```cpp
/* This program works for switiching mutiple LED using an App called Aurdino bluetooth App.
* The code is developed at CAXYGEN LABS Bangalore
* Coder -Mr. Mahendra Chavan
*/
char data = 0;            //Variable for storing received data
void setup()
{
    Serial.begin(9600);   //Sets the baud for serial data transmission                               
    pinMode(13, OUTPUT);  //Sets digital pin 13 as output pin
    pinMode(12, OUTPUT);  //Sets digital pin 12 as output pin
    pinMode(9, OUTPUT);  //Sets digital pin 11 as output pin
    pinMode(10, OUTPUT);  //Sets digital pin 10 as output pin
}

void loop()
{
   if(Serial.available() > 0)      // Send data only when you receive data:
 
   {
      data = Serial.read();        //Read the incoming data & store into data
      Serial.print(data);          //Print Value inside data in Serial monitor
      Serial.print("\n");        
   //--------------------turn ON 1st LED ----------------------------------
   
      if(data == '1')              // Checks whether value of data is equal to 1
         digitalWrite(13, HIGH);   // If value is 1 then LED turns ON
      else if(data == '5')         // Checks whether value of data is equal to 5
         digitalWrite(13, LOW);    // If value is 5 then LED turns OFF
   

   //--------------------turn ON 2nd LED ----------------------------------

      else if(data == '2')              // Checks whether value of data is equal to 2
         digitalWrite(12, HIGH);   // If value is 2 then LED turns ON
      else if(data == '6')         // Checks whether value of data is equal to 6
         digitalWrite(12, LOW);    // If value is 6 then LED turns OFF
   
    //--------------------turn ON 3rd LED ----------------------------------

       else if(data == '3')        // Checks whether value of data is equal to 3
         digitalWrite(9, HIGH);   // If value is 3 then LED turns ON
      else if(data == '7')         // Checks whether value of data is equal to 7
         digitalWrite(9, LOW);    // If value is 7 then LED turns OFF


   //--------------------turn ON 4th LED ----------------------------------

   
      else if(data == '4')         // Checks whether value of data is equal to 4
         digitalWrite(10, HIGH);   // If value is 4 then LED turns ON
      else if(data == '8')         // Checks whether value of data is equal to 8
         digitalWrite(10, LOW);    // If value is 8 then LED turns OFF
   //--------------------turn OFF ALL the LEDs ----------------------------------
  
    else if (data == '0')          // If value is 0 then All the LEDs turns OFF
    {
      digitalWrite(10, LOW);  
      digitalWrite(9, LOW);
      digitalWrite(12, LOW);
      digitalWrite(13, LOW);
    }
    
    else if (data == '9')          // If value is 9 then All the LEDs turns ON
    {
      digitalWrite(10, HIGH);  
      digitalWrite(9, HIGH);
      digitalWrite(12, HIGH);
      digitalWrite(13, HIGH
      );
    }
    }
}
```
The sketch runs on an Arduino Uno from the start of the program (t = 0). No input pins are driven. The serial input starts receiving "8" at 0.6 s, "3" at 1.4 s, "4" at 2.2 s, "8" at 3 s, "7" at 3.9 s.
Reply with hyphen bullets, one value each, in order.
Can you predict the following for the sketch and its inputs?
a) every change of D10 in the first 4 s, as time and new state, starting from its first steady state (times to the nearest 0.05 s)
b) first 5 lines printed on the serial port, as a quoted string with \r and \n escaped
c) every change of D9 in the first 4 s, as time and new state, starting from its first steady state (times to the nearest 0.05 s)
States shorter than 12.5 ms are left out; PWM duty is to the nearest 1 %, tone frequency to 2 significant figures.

- 0 s low; 2.2 s high; 3 s low
- "8\n3\n4\n8\n7\n"
- 0 s low; 1.4 s high; 3.9 s low
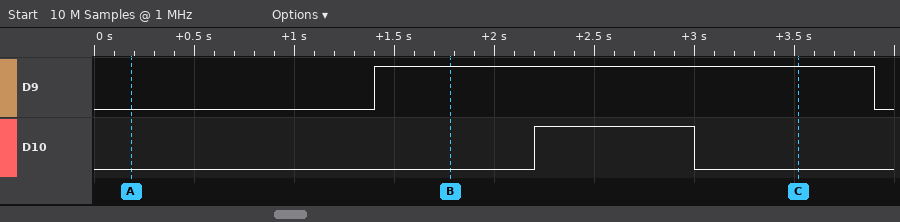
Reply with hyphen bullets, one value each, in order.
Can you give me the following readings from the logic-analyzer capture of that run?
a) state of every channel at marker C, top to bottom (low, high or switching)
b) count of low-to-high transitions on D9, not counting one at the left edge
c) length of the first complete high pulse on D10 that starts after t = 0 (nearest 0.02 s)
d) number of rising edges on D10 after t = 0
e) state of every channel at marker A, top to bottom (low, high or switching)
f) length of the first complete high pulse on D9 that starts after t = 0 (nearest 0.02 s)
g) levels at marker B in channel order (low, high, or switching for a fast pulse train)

- D9 high, D10 low
- 1
- 0.80 s
- 1
- D9 low, D10 low
- 2.50 s
- D9 high, D10 low
